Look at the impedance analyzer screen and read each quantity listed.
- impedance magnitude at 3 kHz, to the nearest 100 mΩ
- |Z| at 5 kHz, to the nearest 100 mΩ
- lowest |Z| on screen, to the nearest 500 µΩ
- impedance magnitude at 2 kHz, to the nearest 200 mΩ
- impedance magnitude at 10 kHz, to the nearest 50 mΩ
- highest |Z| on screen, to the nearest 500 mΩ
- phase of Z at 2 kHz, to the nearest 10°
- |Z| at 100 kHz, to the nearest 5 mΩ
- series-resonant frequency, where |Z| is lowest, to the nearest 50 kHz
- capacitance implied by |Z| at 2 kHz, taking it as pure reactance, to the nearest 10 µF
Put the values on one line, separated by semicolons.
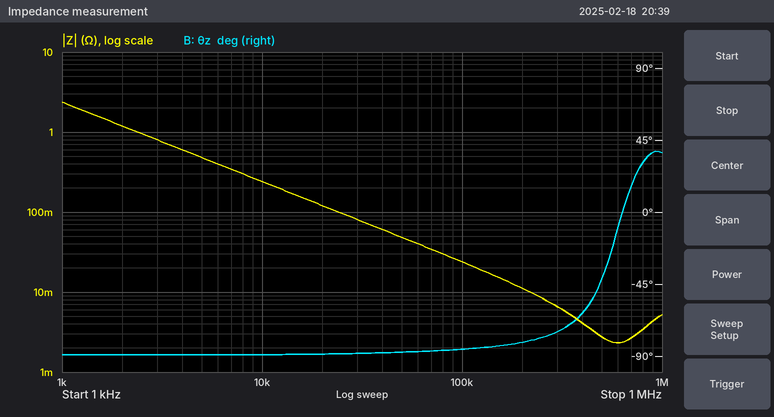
800 mΩ; 500 mΩ; 2.5 mΩ; 1.2 Ω; 250 mΩ; 2.5 Ω; -90°; 25 mΩ; 600 kHz; 70 µF
